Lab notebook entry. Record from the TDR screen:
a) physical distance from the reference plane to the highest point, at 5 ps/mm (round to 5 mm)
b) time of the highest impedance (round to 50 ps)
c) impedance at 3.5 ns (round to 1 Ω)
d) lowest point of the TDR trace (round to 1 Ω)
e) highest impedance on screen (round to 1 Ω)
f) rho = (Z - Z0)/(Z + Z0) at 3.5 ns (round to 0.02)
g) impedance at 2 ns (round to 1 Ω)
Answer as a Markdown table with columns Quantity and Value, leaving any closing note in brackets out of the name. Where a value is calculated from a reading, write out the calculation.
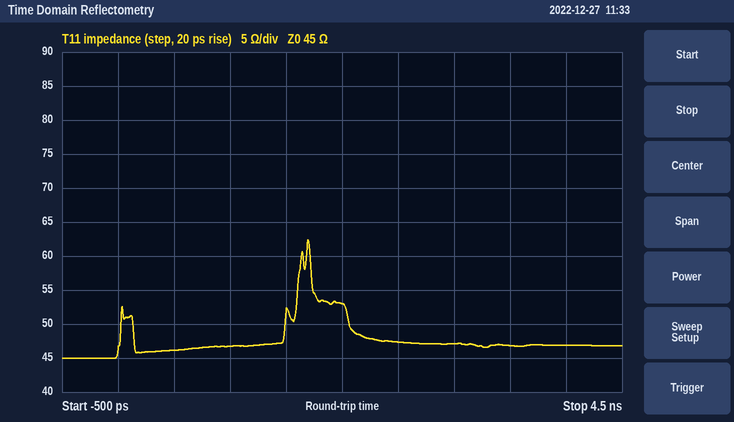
| Quantity | Value |
|---|---|
| physical distance from the reference plane to the highest point, at 5 ps/mm | 1.70 ns / 2 / 5 ps/mm ≈ 170 mm |
| time of the highest impedance | 1.70 ns |
| impedance at 3.5 ns | 47 Ω |
| lowest point of the TDR trace | 45 Ω |
| highest impedance on screen | 62 Ω |
| rho = (Z - Z0)/(Z + Z0) at 3.5 ns | (47 − 45)/(47 + 45) ≈ +0.02 |
| impedance at 2 ns | 53 Ω |
